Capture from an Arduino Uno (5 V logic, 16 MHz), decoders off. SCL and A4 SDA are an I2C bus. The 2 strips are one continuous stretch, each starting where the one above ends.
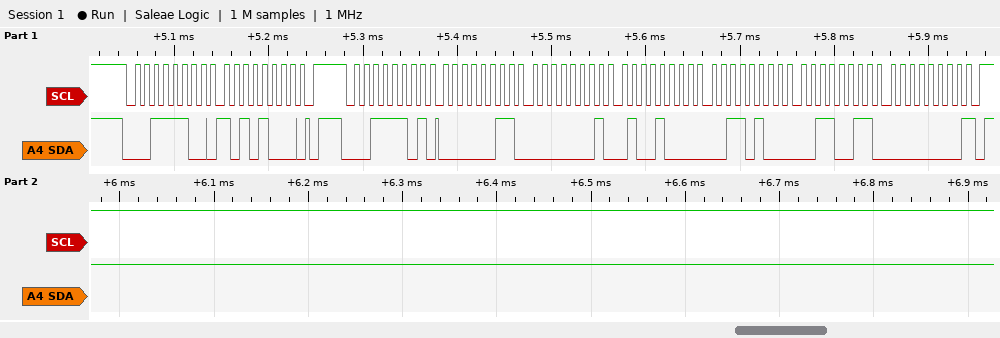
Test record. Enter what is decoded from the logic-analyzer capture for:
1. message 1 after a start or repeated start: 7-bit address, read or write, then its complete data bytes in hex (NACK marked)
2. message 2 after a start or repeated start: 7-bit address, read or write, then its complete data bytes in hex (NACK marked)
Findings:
0x1E write: A8
0x1E read: 03 01 48 34 33 00 NACK
